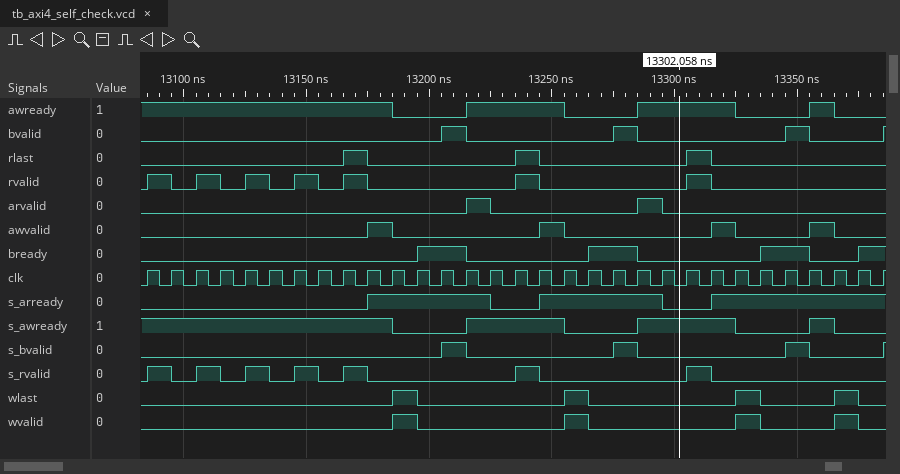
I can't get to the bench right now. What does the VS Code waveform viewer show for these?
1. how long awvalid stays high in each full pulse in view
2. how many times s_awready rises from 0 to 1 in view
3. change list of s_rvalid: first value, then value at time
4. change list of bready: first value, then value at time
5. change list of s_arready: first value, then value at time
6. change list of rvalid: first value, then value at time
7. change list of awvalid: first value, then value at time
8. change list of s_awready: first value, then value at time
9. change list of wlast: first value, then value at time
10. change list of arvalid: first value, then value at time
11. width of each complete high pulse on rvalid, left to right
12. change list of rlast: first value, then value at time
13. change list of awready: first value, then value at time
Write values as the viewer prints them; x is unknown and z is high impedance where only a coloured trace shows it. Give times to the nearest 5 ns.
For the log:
10 ns, 10 ns, 10 ns, 10 ns
3
0, 1 at 13085 ns, 0 at 13095 ns, 1 at 13105 ns, 0 at 13115 ns, 1 at 13125 ns, 0 at 13135 ns, 1 at 13145 ns, 0 at 13155 ns, 1 at 13165 ns, 0 at 13175 ns, 1 at 13235 ns, 0 at 13245 ns, 1 at 13305 ns, 0 at 13315 ns
0, 1 at 13195 ns, 0 at 13215 ns, 1 at 13265 ns, 0 at 13285 ns, 1 at 13335 ns, 0 at 13355 ns, 1 at 13375 ns
0, 1 at 13175 ns, 0 at 13225 ns, 1 at 13245 ns, 0 at 13295 ns, 1 at 13315 ns
0, 1 at 13085 ns, 0 at 13095 ns, 1 at 13105 ns, 0 at 13115 ns, 1 at 13125 ns, 0 at 13135 ns, 1 at 13145 ns, 0 at 13155 ns, 1 at 13165 ns, 0 at 13175 ns, 1 at 13235 ns, 0 at 13245 ns, 1 at 13305 ns, 0 at 13315 ns
0, 1 at 13175 ns, 0 at 13185 ns, 1 at 13245 ns, 0 at 13255 ns, 1 at 13315 ns, 0 at 13325 ns, 1 at 13355 ns, 0 at 13365 ns
1, 0 at 13185 ns, 1 at 13215 ns, 0 at 13255 ns, 1 at 13285 ns, 0 at 13325 ns, 1 at 13355 ns, 0 at 13365 ns
0, 1 at 13185 ns, 0 at 13195 ns, 1 at 13255 ns, 0 at 13265 ns, 1 at 13325 ns, 0 at 13335 ns, 1 at 13365 ns, 0 at 13375 ns
0, 1 at 13215 ns, 0 at 13225 ns, 1 at 13285 ns, 0 at 13295 ns
10 ns, 10 ns, 10 ns, 10 ns, 10 ns, 10 ns, 10 ns
0, 1 at 13165 ns, 0 at 13175 ns, 1 at 13235 ns, 0 at 13245 ns, 1 at 13305 ns, 0 at 13315 ns
1, 0 at 13185 ns, 1 at 13215 ns, 0 at 13255 ns, 1 at 13285 ns, 0 at 13325 ns, 1 at 13355 ns, 0 at 13365 ns
